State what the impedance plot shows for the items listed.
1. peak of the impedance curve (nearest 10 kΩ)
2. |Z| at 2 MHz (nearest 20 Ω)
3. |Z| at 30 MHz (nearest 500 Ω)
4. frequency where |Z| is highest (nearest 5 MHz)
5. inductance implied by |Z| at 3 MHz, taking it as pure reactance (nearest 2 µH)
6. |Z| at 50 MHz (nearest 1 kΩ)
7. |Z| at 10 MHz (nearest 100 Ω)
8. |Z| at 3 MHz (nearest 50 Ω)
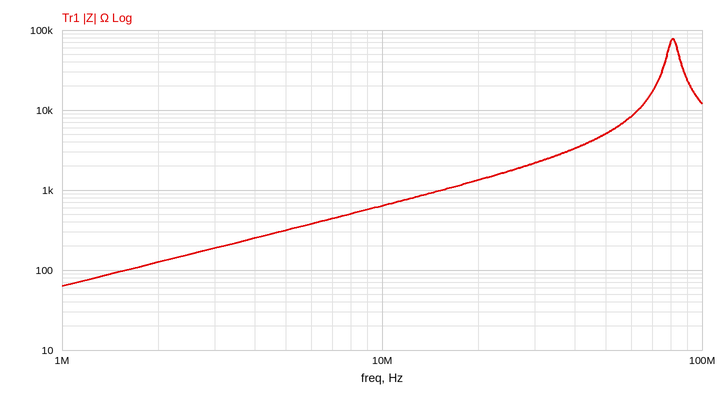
80 kΩ
120 Ω
2.0 kΩ
80 MHz
10 µH
5 kΩ
600 Ω
200 Ω
